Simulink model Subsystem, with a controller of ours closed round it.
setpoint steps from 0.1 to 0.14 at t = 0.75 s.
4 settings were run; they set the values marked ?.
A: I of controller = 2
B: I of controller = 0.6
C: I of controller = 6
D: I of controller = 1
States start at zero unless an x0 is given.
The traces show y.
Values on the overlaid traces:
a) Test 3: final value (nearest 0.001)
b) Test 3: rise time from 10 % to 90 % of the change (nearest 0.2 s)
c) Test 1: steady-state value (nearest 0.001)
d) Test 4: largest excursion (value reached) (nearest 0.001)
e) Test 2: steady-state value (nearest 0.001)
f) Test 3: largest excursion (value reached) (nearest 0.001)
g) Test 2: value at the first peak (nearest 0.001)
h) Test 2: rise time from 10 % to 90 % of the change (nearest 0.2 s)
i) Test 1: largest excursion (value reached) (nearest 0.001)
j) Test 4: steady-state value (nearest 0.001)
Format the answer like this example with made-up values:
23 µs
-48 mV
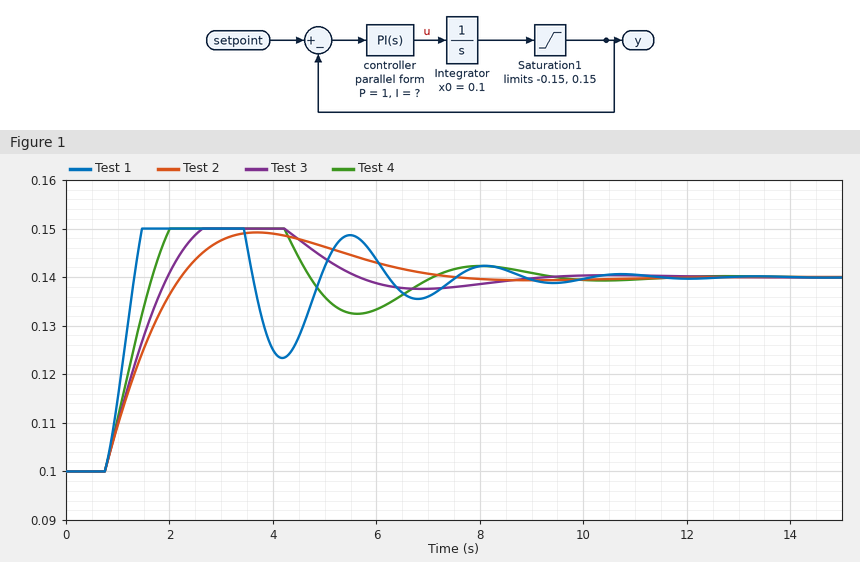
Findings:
0.140
1.0 s
0.140
0.150
0.140
0.150
0.149
1.2 s
0.150
0.140
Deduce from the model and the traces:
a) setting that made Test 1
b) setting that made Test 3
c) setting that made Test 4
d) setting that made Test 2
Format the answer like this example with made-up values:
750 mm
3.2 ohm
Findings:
C
D
A
B
